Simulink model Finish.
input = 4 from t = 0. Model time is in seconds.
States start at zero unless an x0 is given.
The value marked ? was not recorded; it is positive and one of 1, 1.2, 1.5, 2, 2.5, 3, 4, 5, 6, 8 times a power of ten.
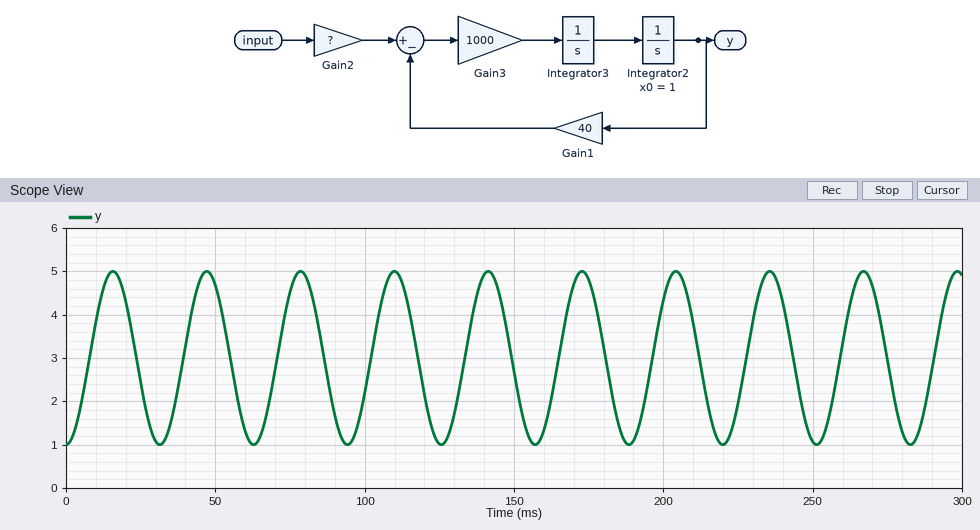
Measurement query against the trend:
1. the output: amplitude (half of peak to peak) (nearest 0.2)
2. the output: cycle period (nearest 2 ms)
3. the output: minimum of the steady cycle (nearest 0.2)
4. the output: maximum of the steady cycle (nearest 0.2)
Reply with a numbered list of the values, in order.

1. 2.0
2. 32 ms
3. 1.0
4. 5.0
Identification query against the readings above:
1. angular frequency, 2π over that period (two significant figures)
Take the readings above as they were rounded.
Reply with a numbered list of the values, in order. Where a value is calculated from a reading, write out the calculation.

1. 2π / 32 = 0.20 rad/ms
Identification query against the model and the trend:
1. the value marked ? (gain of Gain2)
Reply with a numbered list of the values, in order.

1. 30
